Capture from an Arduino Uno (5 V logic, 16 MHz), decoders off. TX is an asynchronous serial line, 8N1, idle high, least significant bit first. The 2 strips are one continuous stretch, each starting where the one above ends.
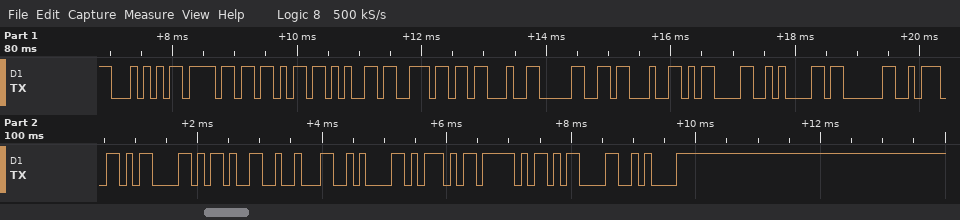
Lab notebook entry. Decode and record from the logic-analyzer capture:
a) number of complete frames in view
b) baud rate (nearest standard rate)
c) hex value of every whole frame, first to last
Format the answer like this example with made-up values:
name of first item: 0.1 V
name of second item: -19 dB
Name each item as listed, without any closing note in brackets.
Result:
number of complete frames in view: 20
baud rate: 9600 baud
hex value of every whole frame, first to last: 54 6F 6B 65 6E 23 30 23 0D 0A 03 3A 0D 2D 12 0A 5D 5F 0D 0A
